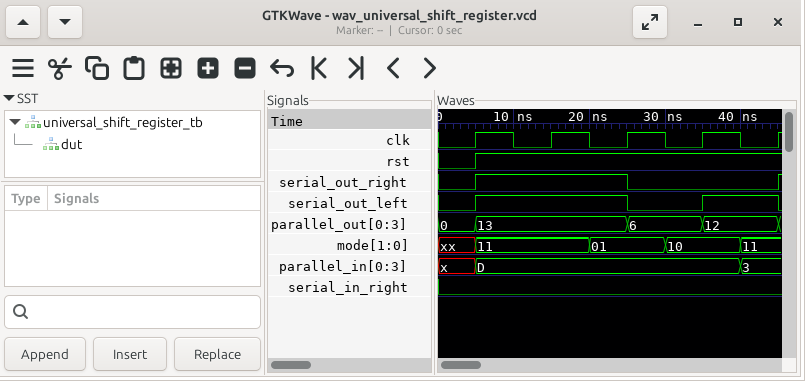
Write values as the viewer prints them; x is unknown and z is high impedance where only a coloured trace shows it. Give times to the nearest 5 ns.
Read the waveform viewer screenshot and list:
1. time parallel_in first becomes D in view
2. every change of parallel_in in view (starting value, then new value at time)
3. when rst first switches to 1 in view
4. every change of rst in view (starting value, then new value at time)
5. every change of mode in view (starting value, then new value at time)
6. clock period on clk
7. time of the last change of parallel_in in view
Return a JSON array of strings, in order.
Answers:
["5 ns", "x, D at 5 ns, 3 at 40 ns", "5 ns", "0, 1 at 5 ns", "xx, 11 at 5 ns, 01 at 20 ns, 10 at 30 ns, 11 at 40 ns", "10 ns", "40 ns"]
